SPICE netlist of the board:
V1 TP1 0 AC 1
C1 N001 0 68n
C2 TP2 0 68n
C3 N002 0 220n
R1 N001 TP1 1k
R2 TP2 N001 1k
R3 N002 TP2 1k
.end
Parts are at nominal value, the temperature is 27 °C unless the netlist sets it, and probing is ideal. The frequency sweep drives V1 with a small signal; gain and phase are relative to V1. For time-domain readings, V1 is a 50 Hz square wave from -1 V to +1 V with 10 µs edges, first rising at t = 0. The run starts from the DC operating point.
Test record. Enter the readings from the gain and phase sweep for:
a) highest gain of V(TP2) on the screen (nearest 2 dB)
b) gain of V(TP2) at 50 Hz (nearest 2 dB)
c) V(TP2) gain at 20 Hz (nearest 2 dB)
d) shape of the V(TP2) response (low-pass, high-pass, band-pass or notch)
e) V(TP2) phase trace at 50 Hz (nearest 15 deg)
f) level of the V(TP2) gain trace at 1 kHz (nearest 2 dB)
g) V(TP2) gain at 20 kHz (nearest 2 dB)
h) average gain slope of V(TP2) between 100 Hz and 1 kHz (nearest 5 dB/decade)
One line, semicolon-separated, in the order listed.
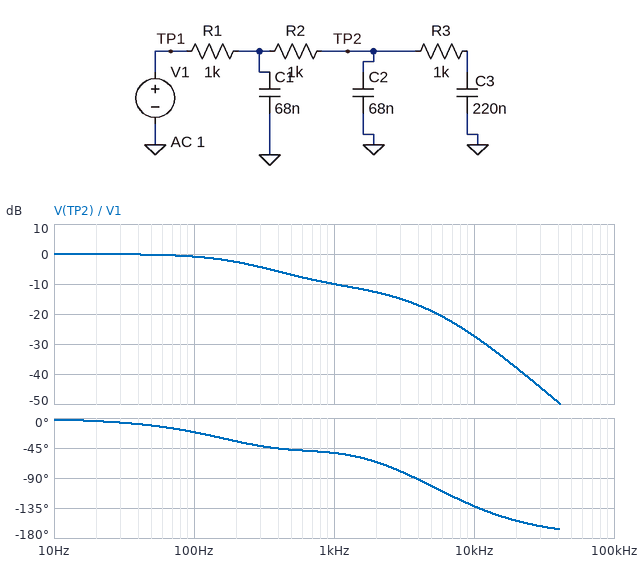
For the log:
0 dB; 0 dB; 0 dB; low-pass; -15 deg; -10 dB; -38 dB; -10 dB/decade
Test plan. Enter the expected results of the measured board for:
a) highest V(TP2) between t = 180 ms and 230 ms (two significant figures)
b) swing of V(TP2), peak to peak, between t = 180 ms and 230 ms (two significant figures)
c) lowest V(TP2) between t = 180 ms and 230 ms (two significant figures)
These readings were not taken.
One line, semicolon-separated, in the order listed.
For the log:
1.0 V; 2.0 V; -1.0 V
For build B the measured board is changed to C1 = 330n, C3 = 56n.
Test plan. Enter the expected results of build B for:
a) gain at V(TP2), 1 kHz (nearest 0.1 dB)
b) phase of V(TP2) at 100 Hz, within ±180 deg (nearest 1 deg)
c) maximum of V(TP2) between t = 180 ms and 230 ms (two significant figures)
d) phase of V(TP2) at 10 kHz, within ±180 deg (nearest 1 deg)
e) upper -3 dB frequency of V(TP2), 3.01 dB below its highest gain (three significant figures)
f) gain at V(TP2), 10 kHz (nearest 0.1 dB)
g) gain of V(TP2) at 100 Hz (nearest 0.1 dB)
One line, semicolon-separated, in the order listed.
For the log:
-11.6 dB; -20 deg; 1.0 V; -152 deg; 305 Hz; -40.3 dB; -0.4 dB
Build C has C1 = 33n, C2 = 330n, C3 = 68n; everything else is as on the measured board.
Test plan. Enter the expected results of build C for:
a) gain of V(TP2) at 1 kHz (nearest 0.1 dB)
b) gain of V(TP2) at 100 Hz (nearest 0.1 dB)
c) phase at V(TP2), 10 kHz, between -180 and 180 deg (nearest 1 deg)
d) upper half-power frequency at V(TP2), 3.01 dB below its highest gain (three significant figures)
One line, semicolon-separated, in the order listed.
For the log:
-14.3 dB; -1.0 dB; -131 deg; 193 Hz
